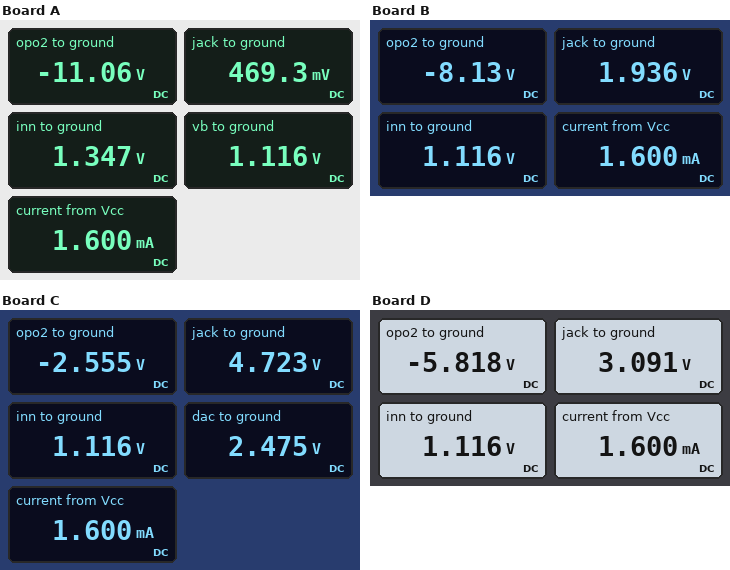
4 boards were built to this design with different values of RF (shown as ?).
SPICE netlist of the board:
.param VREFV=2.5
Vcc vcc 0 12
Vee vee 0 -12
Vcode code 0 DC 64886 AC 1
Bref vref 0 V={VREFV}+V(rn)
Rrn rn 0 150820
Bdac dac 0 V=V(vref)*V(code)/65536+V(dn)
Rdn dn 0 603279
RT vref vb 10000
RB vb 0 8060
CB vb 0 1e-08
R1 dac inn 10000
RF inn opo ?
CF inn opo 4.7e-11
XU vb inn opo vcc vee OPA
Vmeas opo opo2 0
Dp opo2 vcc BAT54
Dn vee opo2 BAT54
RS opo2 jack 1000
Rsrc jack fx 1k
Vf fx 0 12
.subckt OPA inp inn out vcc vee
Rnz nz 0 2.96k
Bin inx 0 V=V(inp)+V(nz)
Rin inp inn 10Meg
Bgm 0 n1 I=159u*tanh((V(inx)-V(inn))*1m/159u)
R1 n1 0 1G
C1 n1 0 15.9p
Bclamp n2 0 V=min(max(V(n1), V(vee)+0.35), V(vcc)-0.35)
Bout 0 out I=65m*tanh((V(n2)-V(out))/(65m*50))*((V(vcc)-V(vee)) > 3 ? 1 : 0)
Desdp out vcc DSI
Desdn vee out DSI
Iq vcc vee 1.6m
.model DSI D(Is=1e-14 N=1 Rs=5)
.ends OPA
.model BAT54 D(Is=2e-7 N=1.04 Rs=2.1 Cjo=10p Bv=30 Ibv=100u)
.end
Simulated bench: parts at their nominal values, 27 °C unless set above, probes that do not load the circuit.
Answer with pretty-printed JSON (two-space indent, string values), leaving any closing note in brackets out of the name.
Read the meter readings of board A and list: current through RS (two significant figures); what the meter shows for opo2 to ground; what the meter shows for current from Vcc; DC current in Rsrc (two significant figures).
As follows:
{
  "current through RS": "12 mA",
  "what the meter shows for opo2 to ground": "-11.06 V",
  "what the meter shows for current from Vcc": "1.600 mA",
  "DC current in Rsrc": "12 mA"
}
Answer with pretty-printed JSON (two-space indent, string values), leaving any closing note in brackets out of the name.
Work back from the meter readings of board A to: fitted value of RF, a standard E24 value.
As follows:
{
  "fitted value of RF, a standard E24 value": "110 kΩ"
}
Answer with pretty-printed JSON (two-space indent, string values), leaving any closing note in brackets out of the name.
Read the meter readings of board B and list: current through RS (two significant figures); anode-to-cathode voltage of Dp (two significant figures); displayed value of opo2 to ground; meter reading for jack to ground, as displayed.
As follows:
{
  "current through RS": "10 mA",
  "anode-to-cathode voltage of Dp": "-20 V",
  "displayed value of opo2 to ground": "-8.13 V",
  "meter reading for jack to ground, as displayed": "1.936 V"
}
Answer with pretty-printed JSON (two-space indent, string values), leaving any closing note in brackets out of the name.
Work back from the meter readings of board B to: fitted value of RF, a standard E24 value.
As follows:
{
  "fitted value of RF, a standard E24 value": "68 kΩ"
}
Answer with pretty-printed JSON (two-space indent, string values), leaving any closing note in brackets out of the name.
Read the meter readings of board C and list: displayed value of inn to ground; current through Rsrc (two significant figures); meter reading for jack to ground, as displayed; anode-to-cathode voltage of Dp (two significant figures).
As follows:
{
  "displayed value of inn to ground": "1.116 V",
  "current through Rsrc": "7.3 mA",
  "meter reading for jack to ground, as displayed": "4.723 V",
  "anode-to-cathode voltage of Dp": "-15 V"
}
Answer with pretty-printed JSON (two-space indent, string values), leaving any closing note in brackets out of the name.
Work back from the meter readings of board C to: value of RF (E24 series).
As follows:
{
  "value of RF": "27 kΩ"
}
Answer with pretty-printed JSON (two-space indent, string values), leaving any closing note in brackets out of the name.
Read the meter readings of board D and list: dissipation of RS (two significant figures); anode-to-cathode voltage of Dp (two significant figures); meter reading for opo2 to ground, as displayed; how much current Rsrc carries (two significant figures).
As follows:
{
  "dissipation of RS": "79 mW",
  "anode-to-cathode voltage of Dp": "-18 V",
  "meter reading for opo2 to ground, as displayed": "-5.818 V",
  "how much current Rsrc carries": "8.9 mA"
}
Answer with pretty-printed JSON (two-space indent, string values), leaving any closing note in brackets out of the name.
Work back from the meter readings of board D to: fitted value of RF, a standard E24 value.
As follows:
{
  "fitted value of RF, a standard E24 value": "51 kΩ"
}
